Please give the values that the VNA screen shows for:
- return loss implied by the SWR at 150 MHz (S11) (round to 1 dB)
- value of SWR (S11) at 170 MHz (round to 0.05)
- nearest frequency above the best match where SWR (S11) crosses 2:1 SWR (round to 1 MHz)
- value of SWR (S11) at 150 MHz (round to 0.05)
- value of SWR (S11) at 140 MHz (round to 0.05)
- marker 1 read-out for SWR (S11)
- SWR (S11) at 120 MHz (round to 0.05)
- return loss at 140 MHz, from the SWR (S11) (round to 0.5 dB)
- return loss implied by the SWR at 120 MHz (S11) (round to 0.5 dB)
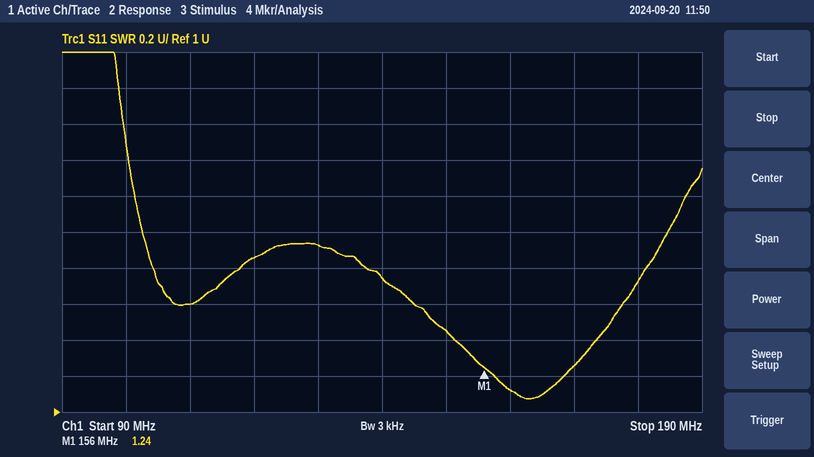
15 dB
1.25
185 MHz
1.45
1.75
1.24
1.85
11.5 dB
10.5 dB
